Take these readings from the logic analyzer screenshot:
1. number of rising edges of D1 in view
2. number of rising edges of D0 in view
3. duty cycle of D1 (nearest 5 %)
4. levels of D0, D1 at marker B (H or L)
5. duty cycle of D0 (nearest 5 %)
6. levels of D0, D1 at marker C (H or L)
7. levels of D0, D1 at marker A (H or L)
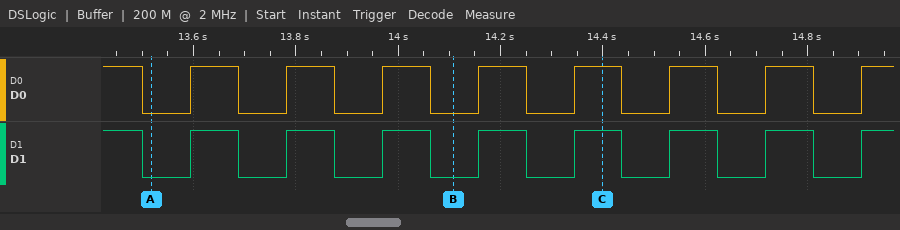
8
8
50 %
D0=L, D1=L
50 %
D0=H, D1=H
D0=L, D1=L
